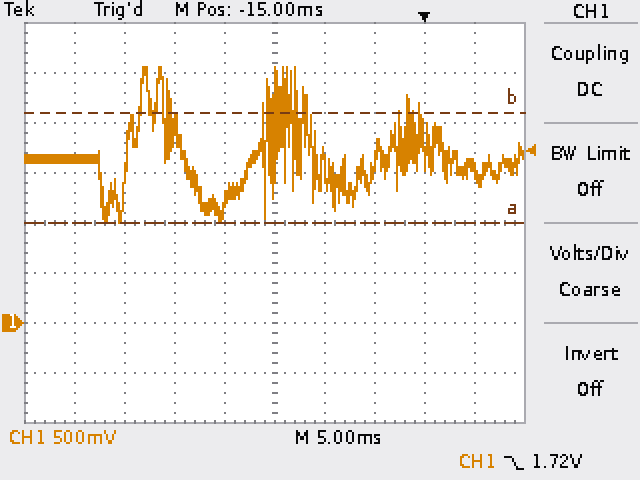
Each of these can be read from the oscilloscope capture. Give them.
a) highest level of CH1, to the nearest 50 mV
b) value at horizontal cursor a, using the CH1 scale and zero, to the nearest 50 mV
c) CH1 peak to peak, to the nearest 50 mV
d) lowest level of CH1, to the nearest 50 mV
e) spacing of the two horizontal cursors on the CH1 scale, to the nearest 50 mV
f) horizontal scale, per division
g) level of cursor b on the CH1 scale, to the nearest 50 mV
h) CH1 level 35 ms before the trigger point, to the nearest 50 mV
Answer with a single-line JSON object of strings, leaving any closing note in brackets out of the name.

{"highest level of CH1, to the nearest 50 mV": "2.55 V", "value at horizontal cursor a, using the CH1 scale and zero, to the nearest 50 mV": "1.00 V", "CH1 peak to peak, to the nearest 50 mV": "1.55 V", "lowest level of CH1, to the nearest 50 mV": "1.00 V", "spacing of the two horizontal cursors on the CH1 scale, to the nearest 50 mV": "1.10 V", "horizontal scale, per division": "5 ms", "level of cursor b on the CH1 scale, to the nearest 50 mV": "2.10 V", "CH1 level 35 ms before the trigger point, to the nearest 50 mV": "1.65 V"}
